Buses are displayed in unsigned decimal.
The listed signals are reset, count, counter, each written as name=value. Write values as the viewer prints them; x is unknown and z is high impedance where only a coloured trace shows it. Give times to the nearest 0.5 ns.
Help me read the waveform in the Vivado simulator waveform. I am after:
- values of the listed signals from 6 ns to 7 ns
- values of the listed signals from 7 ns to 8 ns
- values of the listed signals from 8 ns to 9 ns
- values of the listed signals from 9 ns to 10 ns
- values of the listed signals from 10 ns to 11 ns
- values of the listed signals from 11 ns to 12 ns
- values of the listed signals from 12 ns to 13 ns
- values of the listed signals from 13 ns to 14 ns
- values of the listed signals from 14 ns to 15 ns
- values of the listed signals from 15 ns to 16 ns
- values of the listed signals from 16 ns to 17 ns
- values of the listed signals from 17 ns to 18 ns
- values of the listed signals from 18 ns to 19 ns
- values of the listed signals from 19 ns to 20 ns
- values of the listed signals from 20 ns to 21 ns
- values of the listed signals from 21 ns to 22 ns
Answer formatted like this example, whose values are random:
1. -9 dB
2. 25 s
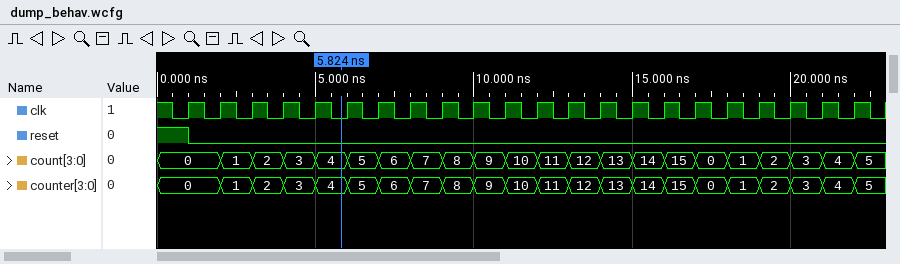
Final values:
1. reset=0, count=5, counter=5
2. reset=0, count=6, counter=6
3. reset=0, count=7, counter=7
4. reset=0, count=8, counter=8
5. reset=0, count=9, counter=9
6. reset=0, count=10, counter=10
7. reset=0, count=11, counter=11
8. reset=0, count=12, counter=12
9. reset=0, count=13, counter=13
10. reset=0, count=14, counter=14
11. reset=0, count=15, counter=15
12. reset=0, count=0, counter=0
13. reset=0, count=1, counter=1
14. reset=0, count=2, counter=2
15. reset=0, count=3, counter=3
16. reset=0, count=4, counter=4
